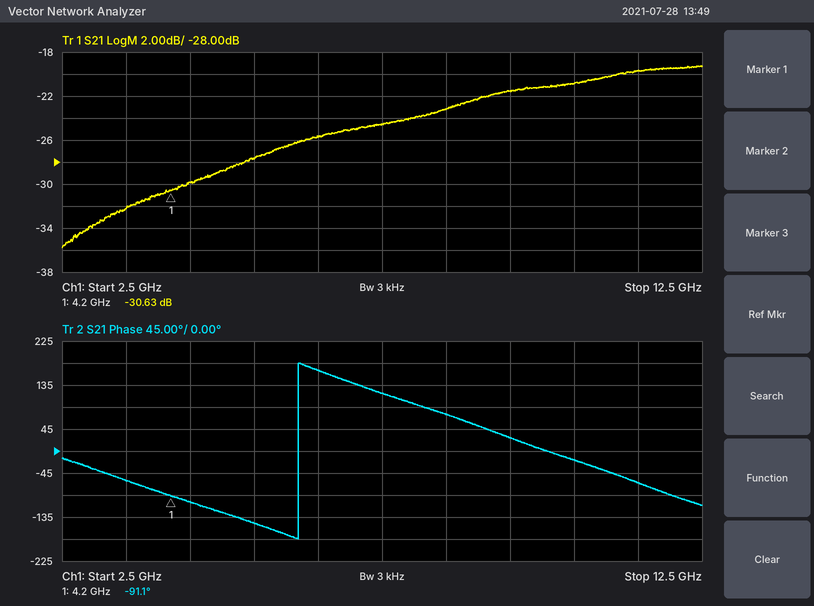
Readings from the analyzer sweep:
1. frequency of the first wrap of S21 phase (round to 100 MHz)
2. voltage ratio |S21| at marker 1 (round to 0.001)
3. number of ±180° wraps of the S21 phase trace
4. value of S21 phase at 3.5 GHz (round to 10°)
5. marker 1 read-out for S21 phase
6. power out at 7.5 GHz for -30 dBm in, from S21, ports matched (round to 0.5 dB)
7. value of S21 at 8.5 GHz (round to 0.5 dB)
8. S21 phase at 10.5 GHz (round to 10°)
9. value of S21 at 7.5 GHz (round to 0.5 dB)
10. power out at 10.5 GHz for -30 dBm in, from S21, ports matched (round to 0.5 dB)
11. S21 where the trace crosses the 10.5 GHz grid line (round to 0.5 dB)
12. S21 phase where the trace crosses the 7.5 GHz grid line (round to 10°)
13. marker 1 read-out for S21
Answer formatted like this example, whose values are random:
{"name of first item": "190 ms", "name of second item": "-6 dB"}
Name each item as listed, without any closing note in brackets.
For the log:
{"frequency of the first wrap of S21 phase": "6.2 GHz", "voltage ratio |S21| at marker 1": "0.029", "number of ±180° wraps of the S21 phase trace": "1", "value of S21 phase at 3.5 GHz": "-60°", "marker 1 read-out for S21 phase": "-91.1°", "power out at 7.5 GHz for -30 dBm in, from S21, ports matched": "-54.5 dBm", "value of S21 at 8.5 GHz": "-23.0 dB", "S21 phase at 10.5 GHz": "-20°", "value of S21 at 7.5 GHz": "-24.5 dB", "power out at 10.5 GHz for -30 dBm in, from S21, ports matched": "-51.0 dBm", "S21 where the trace crosses the 10.5 GHz grid line": "-21.0 dB", "S21 phase where the trace crosses the 7.5 GHz grid line": "120°", "marker 1 read-out for S21": "-30.63 dB"}
